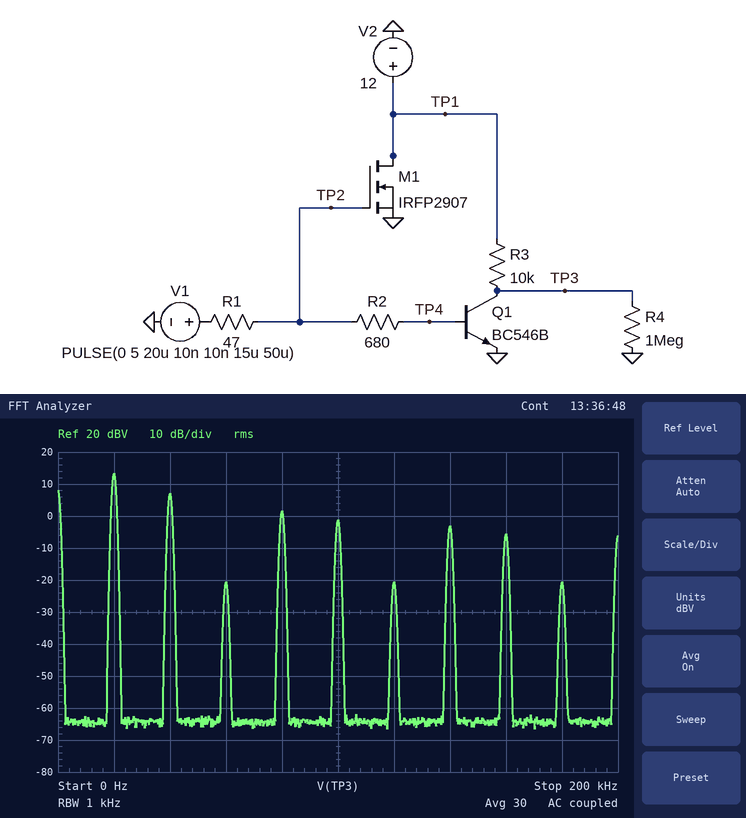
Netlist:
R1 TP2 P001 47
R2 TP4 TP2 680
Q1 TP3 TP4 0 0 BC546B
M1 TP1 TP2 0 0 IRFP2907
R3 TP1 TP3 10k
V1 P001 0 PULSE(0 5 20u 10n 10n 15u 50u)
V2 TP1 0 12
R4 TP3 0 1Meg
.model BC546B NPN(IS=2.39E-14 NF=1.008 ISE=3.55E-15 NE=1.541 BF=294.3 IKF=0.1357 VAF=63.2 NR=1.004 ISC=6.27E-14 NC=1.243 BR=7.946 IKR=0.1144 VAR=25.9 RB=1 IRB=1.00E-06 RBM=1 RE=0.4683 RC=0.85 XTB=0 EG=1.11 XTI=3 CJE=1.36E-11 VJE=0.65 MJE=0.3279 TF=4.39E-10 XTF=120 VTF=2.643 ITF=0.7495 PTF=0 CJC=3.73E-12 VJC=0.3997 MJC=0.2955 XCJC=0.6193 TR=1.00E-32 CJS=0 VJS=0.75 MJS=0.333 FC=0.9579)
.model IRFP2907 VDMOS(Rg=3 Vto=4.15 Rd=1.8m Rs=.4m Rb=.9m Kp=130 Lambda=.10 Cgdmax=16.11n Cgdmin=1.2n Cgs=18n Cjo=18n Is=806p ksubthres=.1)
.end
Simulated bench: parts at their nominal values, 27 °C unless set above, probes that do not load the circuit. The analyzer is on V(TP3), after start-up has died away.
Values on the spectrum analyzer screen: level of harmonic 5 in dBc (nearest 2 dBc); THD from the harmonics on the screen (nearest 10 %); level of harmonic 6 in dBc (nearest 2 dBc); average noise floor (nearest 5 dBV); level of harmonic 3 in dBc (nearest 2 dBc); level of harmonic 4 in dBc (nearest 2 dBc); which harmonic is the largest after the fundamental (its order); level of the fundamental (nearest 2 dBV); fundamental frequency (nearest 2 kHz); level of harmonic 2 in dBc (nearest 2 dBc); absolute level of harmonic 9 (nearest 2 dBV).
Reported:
-14 dBc
60 %
-34 dBc
-65 dBV
-34 dBc
-12 dBc
2
14 dBV
20 kHz
-6 dBc
-20 dBV
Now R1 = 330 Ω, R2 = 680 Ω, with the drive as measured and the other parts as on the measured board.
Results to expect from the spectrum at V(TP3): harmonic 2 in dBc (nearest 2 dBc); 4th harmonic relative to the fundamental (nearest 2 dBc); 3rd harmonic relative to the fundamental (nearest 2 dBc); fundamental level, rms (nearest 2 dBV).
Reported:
-22 dBc
-22 dBc
-10 dBc
14 dBV
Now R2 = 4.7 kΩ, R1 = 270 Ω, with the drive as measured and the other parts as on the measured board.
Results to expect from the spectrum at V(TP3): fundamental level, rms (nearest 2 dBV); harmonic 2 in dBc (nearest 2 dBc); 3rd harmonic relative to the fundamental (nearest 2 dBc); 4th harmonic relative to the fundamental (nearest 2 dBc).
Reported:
14 dBV
-36 dBc
-10 dBc
-36 dBc
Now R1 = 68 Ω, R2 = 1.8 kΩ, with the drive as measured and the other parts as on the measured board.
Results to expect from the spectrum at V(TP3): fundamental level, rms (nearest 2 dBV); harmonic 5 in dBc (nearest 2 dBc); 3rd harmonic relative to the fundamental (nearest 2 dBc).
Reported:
14 dBV
-18 dBc
-22 dBc
